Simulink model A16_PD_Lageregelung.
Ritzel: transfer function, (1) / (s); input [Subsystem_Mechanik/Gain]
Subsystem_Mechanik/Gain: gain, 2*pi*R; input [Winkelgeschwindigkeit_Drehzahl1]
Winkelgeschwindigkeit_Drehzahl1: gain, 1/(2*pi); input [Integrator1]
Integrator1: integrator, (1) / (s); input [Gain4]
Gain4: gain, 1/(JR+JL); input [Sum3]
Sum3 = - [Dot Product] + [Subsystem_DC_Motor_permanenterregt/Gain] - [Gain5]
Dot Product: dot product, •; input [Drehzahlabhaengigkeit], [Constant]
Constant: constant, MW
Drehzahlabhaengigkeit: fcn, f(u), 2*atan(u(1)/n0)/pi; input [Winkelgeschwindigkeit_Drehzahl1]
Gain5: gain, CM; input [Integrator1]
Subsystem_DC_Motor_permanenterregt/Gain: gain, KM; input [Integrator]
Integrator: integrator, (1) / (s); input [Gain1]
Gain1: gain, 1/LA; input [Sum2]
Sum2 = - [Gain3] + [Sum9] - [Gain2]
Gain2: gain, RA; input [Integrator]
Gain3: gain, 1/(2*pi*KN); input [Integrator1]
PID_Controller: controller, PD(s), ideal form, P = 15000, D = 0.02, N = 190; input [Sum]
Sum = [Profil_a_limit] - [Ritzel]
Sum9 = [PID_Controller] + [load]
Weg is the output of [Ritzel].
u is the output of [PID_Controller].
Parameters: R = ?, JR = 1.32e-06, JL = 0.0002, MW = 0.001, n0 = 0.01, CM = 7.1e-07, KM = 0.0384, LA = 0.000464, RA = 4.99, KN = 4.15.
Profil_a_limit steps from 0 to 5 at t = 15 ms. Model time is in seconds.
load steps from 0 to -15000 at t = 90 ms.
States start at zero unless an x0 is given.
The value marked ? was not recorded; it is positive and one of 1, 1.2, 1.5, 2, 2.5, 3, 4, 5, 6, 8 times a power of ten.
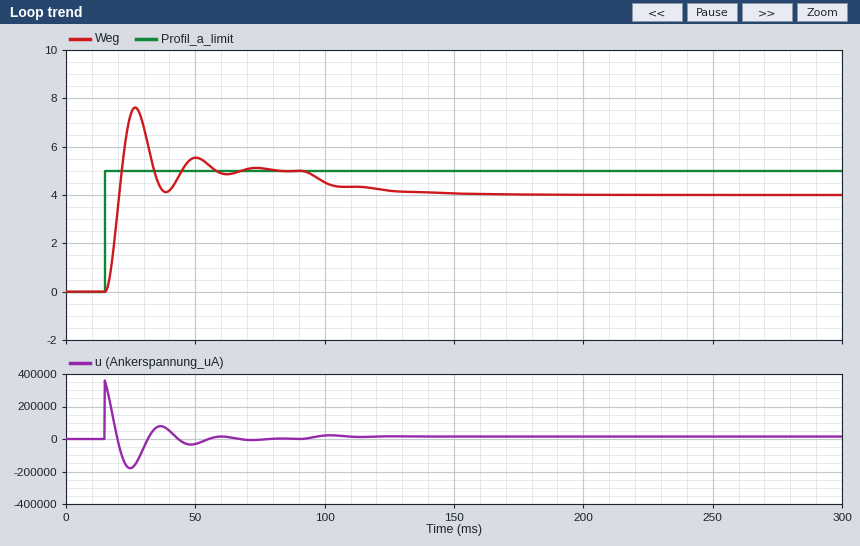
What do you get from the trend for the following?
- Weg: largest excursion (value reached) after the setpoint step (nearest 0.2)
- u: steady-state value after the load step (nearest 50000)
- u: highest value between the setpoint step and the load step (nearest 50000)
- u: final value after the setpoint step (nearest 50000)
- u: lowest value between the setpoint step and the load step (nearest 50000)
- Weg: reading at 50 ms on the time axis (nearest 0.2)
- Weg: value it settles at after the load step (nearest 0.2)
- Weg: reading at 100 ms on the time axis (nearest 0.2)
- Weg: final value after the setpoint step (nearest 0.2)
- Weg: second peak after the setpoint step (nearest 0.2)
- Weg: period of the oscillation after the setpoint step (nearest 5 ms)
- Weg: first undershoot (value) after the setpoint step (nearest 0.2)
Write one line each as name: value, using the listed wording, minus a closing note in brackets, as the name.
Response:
Weg: largest excursion (value reached) after the setpoint step: 7.6
u: steady-state value after the load step: 0
u: highest value between the setpoint step and the load step: 350000
u: final value after the setpoint step: 0
u: lowest value between the setpoint step and the load step: -200000
Weg: reading at 50 ms on the time axis: 5.6
Weg: value it settles at after the load step: 4.0
Weg: reading at 100 ms on the time axis: 4.6
Weg: final value after the setpoint step: 5.0
Weg: second peak after the setpoint step: 5.6
Weg: period of the oscillation after the setpoint step: 25 ms
Weg: first undershoot (value) after the setpoint step: 4.2
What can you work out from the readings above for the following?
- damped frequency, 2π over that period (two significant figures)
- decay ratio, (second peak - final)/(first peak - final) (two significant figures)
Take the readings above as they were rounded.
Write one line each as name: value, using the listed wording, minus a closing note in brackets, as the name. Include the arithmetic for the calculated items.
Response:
damped frequency, 2π over that period: 2π / 25 = 0.25 rad/ms
decay ratio, (second peak - final)/(first peak - final): (5.6 - 5) / (7.6 - 5) = 0.23
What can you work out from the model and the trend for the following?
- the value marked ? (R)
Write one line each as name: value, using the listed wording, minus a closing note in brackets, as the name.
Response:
the value marked ?: 0.03
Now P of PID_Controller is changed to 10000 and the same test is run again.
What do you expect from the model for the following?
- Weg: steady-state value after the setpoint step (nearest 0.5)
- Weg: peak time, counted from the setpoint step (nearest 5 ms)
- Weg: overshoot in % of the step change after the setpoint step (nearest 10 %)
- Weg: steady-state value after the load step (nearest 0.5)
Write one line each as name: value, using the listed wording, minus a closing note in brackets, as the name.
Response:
Weg: steady-state value after the setpoint step: 5.0
Weg: peak time, counted from the setpoint step: 15 ms
Weg: overshoot in % of the step change after the setpoint step: 50 %
Weg: steady-state value after the load step: 3.5
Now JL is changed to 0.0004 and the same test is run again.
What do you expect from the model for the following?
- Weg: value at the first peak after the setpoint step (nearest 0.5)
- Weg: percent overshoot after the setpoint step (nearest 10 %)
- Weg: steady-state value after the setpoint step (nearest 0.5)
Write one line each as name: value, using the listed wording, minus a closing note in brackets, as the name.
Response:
Weg: value at the first peak after the setpoint step: 7.0
Weg: percent overshoot after the setpoint step: 40 %
Weg: steady-state value after the setpoint step: 5.0
